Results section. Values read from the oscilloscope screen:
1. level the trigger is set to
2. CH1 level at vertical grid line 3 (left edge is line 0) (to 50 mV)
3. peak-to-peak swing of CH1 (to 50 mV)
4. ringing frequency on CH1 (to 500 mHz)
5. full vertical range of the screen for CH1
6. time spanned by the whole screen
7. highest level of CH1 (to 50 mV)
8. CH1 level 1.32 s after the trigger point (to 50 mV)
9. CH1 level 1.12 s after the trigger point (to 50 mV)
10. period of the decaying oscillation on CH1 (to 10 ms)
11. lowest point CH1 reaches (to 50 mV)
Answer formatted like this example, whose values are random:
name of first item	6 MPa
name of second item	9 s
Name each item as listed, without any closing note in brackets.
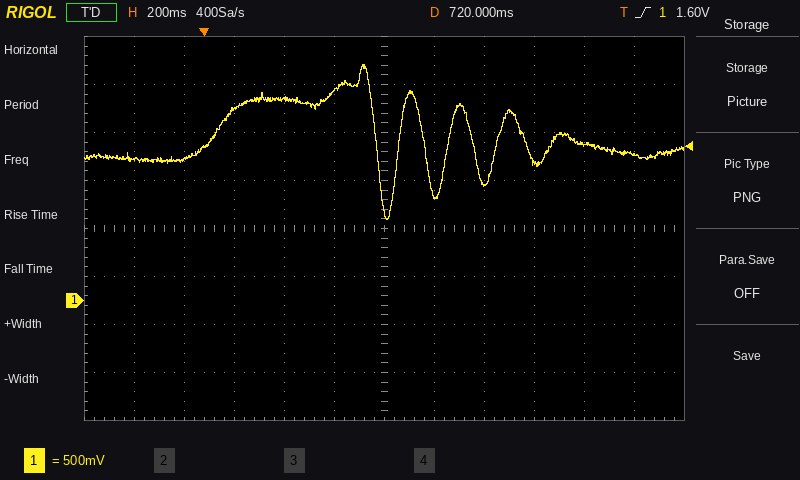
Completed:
level the trigger is set to	1.60 V
CH1 level at vertical grid line 3 (left edge is line 0)	2.00 V
peak-to-peak swing of CH1	1.60 V
ringing frequency on CH1	5.0 Hz
full vertical range of the screen for CH1	4 V
time spanned by the whole screen	2.4 s
highest level of CH1	2.45 V
CH1 level 1.32 s after the trigger point	1.45 V
CH1 level 1.12 s after the trigger point	1.20 V
period of the decaying oscillation on CH1	200 ms
lowest point CH1 reaches	850 mV
